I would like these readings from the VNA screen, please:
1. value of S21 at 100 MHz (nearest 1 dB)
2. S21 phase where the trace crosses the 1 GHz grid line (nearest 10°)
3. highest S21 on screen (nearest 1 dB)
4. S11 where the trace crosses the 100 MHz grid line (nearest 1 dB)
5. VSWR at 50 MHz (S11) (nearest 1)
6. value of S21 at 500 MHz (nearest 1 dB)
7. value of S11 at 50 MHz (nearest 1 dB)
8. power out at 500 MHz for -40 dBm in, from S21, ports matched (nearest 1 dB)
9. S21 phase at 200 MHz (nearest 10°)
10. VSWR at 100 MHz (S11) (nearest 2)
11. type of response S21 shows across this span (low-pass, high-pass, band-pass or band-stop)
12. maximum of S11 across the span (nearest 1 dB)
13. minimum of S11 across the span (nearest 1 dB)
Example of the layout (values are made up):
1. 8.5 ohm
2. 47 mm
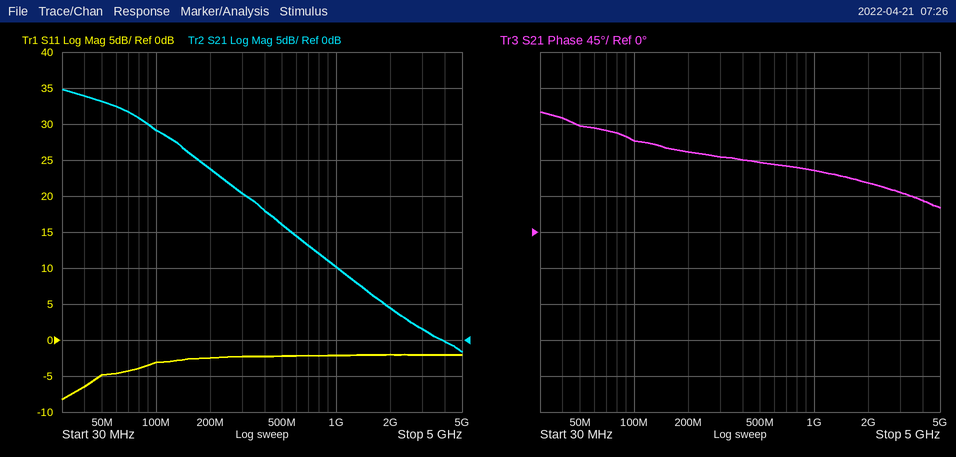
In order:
1. 29 dB
2. 80°
3. 35 dB
4. -3 dB
5. 4
6. 16 dB
7. -5 dB
8. -24 dBm
9. 100°
10. 6
11. low-pass
12. -2 dB
13. -8 dB
